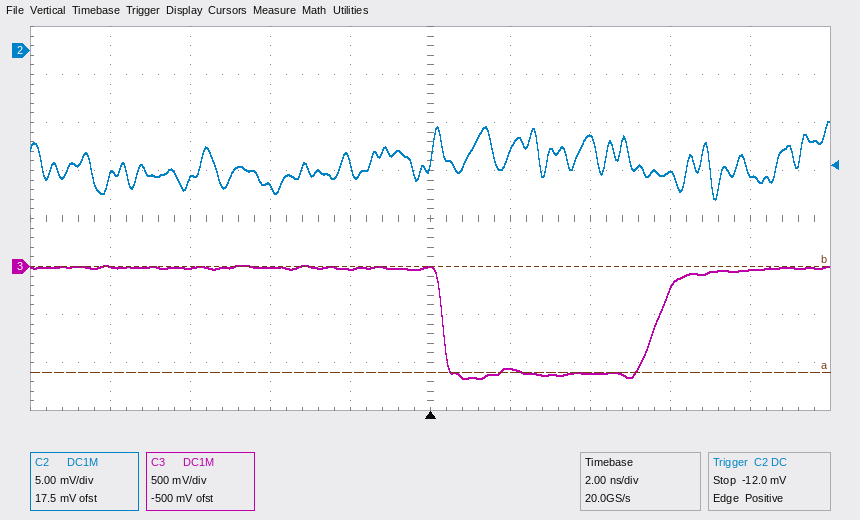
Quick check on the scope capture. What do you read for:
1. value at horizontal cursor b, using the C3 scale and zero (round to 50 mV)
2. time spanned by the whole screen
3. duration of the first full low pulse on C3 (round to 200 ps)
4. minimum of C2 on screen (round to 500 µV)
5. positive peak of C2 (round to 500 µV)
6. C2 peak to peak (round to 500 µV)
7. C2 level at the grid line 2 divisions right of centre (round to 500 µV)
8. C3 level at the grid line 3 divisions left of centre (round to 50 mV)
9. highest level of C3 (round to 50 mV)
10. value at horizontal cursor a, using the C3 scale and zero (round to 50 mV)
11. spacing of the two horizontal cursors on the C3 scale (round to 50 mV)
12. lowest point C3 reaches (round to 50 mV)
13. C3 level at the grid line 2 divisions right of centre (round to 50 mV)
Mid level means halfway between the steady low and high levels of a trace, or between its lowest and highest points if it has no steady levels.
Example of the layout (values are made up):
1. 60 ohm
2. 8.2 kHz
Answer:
1. 0 mV
2. 20 ns
3. 5.4 ns
4. -15.5 mV
5. -7.5 mV
6. 8.0 mV
7. -9.0 mV
8. 0 mV
9. 0 mV
10. -1.10 V
11. 1.10 V
12. -1.15 V
13. -1.10 V
